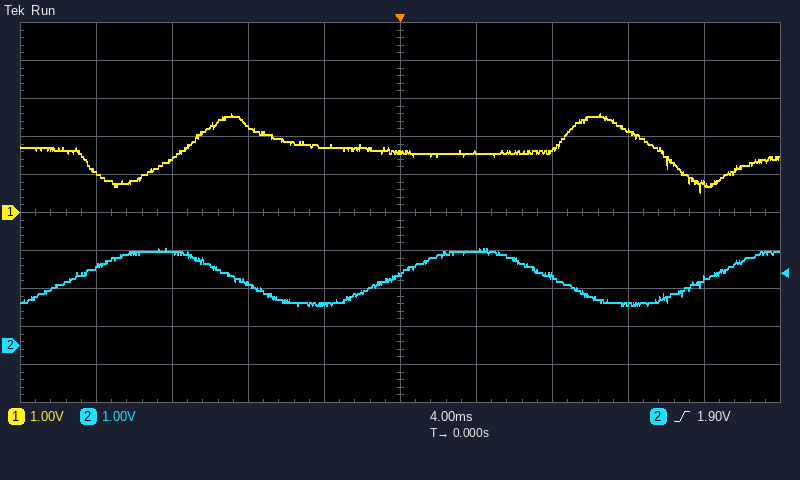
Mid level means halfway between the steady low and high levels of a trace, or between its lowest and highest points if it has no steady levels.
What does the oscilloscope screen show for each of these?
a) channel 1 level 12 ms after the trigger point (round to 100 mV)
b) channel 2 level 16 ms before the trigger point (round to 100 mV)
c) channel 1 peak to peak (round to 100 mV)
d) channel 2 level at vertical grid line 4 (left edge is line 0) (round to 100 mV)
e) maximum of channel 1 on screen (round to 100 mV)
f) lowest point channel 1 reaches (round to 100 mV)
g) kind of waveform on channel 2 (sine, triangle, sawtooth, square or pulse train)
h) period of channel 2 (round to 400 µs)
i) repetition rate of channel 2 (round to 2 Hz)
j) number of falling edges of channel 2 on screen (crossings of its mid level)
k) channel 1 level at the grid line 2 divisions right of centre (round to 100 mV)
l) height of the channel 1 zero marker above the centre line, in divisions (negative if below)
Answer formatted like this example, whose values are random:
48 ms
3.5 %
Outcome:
2.1 V
2.1 V
2.1 V
1.1 V
2.6 V
500 mV
sine
16.8 ms
60 Hz
2
1.6 V
0.0 div
